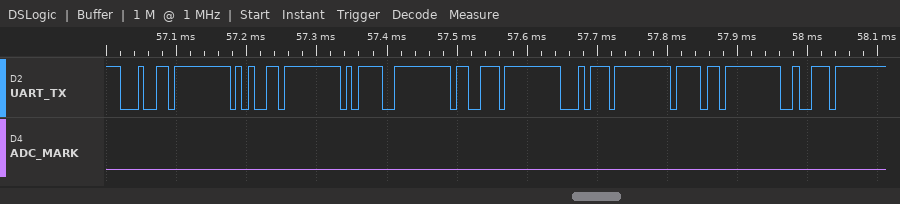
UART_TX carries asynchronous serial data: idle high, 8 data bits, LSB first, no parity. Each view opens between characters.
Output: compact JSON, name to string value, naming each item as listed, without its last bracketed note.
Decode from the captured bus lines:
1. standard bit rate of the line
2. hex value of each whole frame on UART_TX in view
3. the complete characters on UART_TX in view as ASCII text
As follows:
{"standard bit rate of the line": "115200 baud", "hex value of each whole frame on UART_TX in view": "64, 65, 3D, 73, 74, 6F, 72", "the complete characters on UART_TX in view as ASCII text": "\"de=stor\""}
